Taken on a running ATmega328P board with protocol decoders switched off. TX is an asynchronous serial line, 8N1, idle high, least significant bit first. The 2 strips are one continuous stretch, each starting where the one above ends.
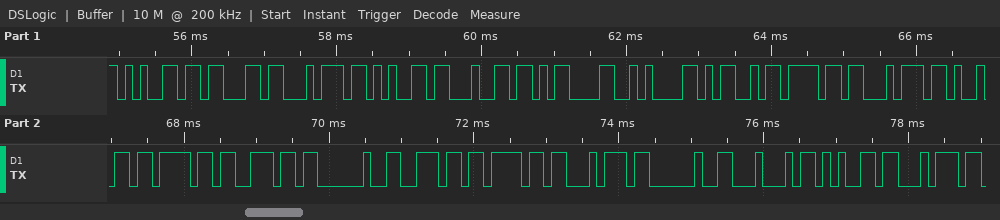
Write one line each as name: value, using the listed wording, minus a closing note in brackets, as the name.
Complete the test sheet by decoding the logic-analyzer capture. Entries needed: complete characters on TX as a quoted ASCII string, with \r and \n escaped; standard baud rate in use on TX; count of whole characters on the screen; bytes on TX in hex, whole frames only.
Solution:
complete characters on TX as a quoted ASCII string, with \r and \n escaped: "ected\r\nMotion not Det"
standard baud rate in use on TX: 9600 baud
count of whole characters on the screen: 21
bytes on TX in hex, whole frames only: 0x65 0x63 0x74 0x65 0x64 0x0D 0x0A 0x4D 0x6F 0x74 0x69 0x6F 0x6E 0x20 0x6E 0x6F 0x74 0x20 0x44 0x65 0x74
